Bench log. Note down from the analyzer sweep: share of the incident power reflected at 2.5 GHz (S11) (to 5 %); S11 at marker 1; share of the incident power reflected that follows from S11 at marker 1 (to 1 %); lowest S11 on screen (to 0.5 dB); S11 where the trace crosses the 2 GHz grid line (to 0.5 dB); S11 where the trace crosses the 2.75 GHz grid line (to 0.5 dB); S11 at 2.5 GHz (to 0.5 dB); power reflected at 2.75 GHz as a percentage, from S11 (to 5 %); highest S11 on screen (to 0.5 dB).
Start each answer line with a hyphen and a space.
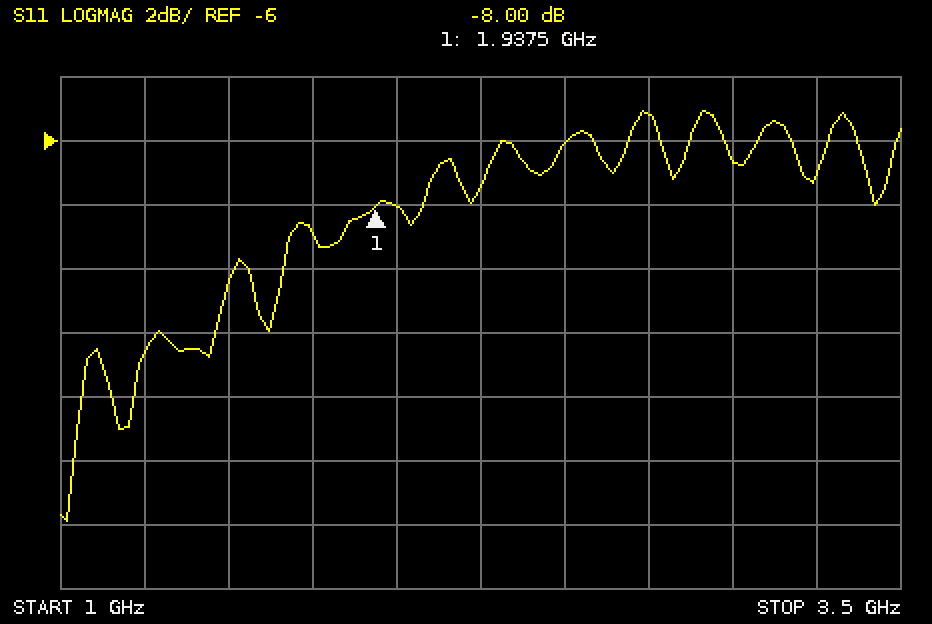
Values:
- 25 %
- -8.00 dB
- 16 %
- -18.0 dB
- -8.0 dB
- -5.0 dB
- -6.0 dB
- 30 %
- -5.0 dB
